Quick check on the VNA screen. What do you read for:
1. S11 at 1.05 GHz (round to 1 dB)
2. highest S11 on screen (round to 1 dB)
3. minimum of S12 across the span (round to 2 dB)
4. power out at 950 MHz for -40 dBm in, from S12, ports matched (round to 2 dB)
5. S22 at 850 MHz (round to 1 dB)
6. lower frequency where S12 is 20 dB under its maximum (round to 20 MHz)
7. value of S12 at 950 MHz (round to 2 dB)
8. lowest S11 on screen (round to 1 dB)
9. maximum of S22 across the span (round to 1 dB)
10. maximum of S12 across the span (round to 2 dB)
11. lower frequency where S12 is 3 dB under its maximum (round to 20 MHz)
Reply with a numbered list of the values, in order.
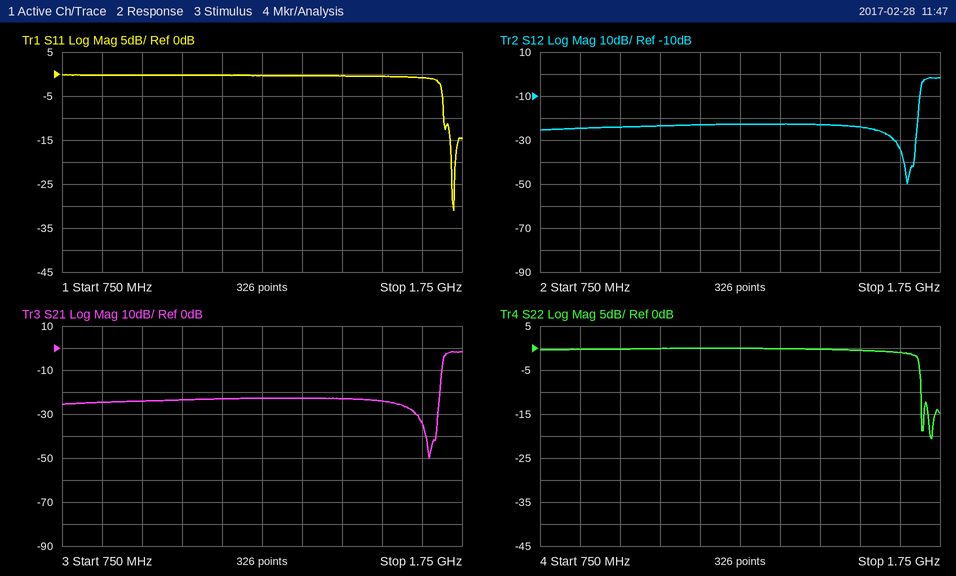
1. 0 dB
2. 0 dB
3. -50 dB
4. -64 dBm
5. 0 dB
6. 1.70 GHz
7. -24 dB
8. -31 dB
9. 0 dB
10. -2 dB
11. 1.70 GHz
